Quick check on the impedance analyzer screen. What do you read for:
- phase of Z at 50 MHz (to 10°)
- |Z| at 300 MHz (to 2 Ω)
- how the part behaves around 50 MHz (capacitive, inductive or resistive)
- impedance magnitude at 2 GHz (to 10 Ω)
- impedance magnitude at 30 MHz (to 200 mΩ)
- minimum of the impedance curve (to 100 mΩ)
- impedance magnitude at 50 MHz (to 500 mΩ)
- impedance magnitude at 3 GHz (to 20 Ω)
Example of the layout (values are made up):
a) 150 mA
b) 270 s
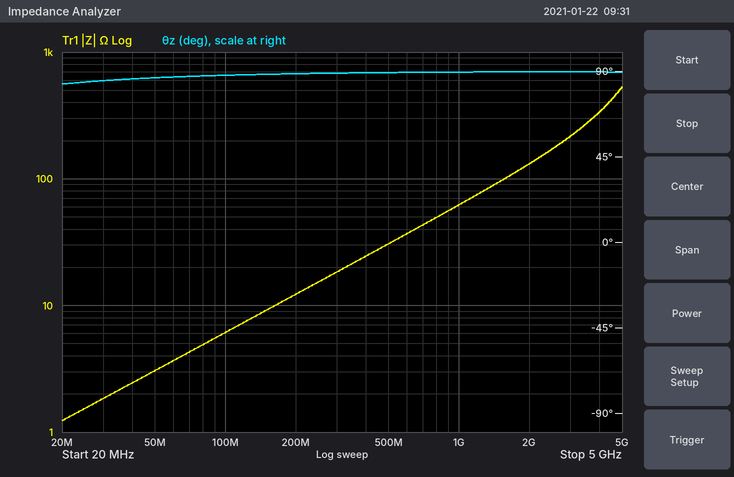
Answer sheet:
a) 90°
b) 18 Ω
c) inductive
d) 130 Ω
e) 1.8 Ω
f) 1.2 Ω
g) 3.0 Ω
h) 220 Ω
